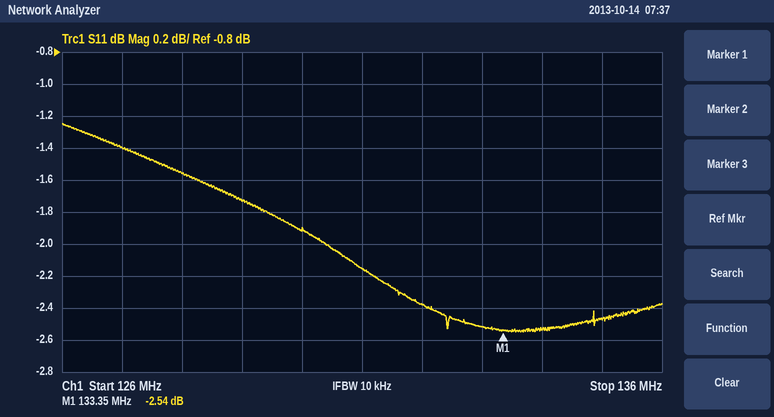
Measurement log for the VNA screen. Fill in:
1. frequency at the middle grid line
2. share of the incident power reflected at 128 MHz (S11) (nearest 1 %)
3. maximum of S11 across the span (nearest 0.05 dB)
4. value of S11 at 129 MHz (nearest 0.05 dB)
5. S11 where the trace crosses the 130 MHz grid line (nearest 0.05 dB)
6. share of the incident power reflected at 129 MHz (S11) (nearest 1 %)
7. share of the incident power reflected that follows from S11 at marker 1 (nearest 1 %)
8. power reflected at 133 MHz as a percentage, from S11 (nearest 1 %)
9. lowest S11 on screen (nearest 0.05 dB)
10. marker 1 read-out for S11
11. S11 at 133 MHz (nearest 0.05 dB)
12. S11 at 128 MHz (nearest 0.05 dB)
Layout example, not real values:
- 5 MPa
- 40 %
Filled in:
- 131 MHz
- 70 %
- -1.25 dB
- -1.75 dB
- -1.90 dB
- 67 %
- 56 %
- 56 %
- -2.55 dB
- -2.54 dB
- -2.50 dB
- -1.55 dB
